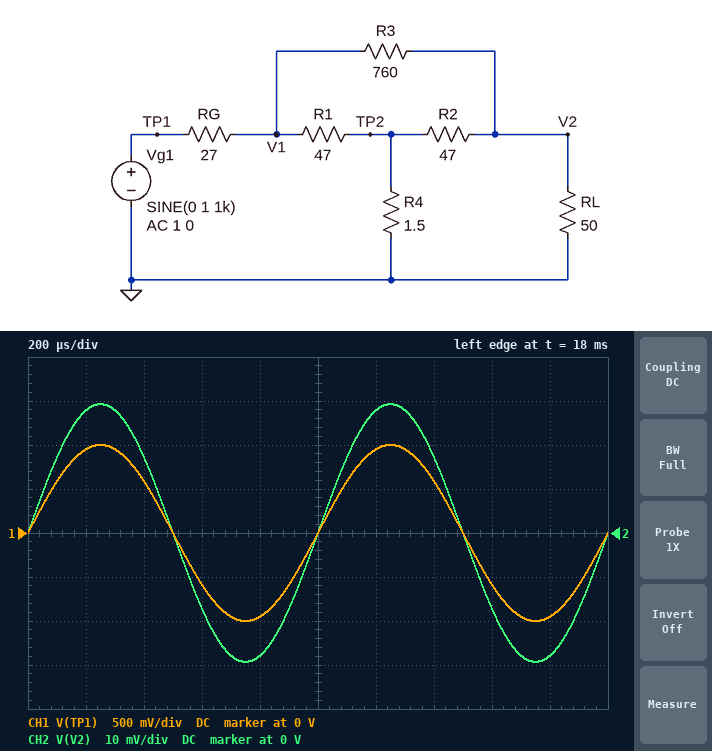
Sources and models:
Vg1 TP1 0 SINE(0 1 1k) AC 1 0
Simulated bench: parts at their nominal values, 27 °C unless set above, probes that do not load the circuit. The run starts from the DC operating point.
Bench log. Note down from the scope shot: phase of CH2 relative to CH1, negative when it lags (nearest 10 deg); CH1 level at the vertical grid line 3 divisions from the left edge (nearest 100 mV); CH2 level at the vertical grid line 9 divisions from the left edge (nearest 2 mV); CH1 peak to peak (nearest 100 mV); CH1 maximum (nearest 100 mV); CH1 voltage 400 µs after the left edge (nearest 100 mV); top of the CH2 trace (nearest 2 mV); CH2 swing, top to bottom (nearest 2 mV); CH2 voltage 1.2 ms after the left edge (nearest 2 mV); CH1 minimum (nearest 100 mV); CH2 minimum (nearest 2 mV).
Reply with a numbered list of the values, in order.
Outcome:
1. 0 deg
2. -600 mV
3. -28 mV
4. 2.0 V
5. 1.0 V
6. 600 mV
7. 30 mV
8. 58 mV
9. 28 mV
10. -1.0 V
11. -30 mV
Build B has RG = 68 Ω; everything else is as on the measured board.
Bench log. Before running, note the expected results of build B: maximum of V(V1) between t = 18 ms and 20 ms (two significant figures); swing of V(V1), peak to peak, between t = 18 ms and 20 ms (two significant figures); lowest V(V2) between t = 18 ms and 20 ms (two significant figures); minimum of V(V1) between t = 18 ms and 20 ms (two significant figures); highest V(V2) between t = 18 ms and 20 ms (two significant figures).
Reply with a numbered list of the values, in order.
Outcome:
1. 400 mV
2. 800 mV
3. -19 mV
4. -400 mV
5. 19 mV
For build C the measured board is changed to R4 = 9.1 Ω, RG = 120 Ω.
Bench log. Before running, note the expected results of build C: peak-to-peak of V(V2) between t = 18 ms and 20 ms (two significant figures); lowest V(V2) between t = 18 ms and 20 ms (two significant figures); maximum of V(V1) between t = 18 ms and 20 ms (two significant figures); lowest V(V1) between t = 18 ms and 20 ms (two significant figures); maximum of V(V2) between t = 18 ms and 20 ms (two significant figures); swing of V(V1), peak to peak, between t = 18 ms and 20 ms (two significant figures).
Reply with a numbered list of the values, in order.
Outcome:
1. 66 mV
2. -33 mV
3. 300 mV
4. -300 mV
5. 33 mV
6. 610 mV
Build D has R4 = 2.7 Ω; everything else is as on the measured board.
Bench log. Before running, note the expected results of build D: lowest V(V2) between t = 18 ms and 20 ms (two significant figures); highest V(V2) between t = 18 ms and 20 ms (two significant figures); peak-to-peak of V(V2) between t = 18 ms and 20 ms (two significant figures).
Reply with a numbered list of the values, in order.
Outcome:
1. -37 mV
2. 37 mV
3. 74 mV
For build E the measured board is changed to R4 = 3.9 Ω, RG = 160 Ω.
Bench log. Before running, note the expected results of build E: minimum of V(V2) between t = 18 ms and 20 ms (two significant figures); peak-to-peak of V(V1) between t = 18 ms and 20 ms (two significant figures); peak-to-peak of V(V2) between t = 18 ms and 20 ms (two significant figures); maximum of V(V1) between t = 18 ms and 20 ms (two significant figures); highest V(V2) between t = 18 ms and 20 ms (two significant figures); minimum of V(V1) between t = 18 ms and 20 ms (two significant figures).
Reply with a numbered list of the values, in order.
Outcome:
1. -16 mV
2. 460 mV
3. 32 mV
4. 230 mV
5. 16 mV
6. -230 mV
